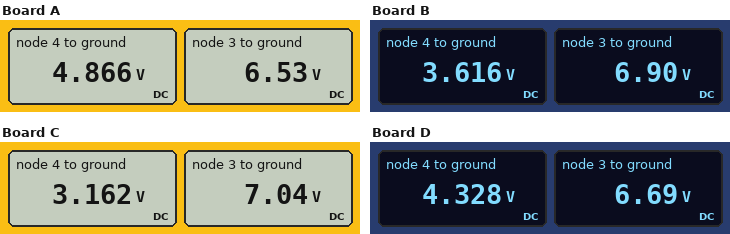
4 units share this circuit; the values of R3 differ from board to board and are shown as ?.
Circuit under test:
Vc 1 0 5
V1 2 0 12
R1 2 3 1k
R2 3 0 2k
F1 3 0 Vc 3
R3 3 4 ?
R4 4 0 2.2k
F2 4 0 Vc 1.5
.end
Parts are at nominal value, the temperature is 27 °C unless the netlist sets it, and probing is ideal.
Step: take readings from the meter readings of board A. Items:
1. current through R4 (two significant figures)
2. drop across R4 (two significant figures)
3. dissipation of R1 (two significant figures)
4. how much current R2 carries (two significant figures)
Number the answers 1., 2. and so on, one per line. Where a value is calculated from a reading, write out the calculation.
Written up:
1. (4.866 V) / 2.2 kΩ = 2.2 mA
2. 4.866 V = 4.9 V
3. (12 V - 6.53 V)^2 / 1 kΩ = 30 mW
4. (6.53 V) / 2 kΩ = 3.3 mA
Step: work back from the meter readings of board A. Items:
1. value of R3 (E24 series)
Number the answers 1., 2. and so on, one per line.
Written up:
1. 750 Ω
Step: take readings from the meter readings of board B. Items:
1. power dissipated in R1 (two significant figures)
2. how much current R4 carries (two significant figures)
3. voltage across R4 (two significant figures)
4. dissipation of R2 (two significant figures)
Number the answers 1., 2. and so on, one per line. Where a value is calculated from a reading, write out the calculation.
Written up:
1. (12 V - 6.9 V)^2 / 1 kΩ = 26 mW
2. (3.616 V) / 2.2 kΩ = 1.6 mA
3. 3.616 V = 3.6 V
4. (6.9 V)^2 / 2 kΩ = 24 mW
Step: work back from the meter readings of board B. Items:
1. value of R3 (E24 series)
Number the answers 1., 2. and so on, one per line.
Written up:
1. 2 kΩ
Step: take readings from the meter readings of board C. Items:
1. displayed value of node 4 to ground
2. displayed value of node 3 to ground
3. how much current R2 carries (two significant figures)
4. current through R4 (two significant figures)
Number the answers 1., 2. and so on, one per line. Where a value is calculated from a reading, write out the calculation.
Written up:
1. 3.162 V
2. 7.04 V
3. (7.04 V) / 2 kΩ = 3.5 mA
4. (3.162 V) / 2.2 kΩ = 1.4 mA
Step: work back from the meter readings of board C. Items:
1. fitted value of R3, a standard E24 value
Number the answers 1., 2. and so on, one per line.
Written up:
1. 2.7 kΩ
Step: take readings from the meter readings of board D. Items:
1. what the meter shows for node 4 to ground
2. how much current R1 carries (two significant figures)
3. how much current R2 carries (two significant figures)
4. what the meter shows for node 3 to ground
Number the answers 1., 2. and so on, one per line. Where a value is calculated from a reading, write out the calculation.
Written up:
1. 4.328 V
2. (12 V - 6.69 V) / 1 kΩ = 5.3 mA
3. (6.69 V) / 2 kΩ = 3.3 mA
4. 6.69 V
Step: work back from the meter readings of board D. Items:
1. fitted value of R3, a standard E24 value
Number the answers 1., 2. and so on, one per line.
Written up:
1. 1.2 kΩ
